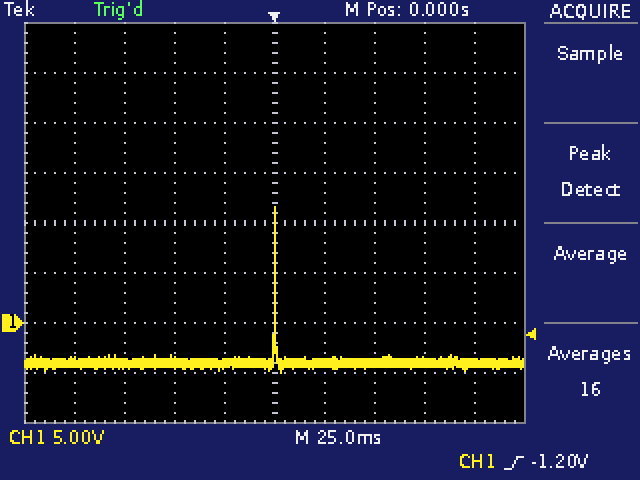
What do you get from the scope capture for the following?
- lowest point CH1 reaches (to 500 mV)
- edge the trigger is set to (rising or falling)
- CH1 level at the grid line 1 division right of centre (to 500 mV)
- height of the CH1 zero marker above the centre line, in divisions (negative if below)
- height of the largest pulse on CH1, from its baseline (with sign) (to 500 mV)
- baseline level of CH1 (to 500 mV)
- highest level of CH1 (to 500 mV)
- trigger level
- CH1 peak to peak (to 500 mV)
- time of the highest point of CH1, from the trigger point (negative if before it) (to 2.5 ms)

-5.0 V
rising
-4.0 V
-2.0 div
+15.5 V
-4.0 V
11.5 V
-1.20 V
16.5 V
0.0 ms
